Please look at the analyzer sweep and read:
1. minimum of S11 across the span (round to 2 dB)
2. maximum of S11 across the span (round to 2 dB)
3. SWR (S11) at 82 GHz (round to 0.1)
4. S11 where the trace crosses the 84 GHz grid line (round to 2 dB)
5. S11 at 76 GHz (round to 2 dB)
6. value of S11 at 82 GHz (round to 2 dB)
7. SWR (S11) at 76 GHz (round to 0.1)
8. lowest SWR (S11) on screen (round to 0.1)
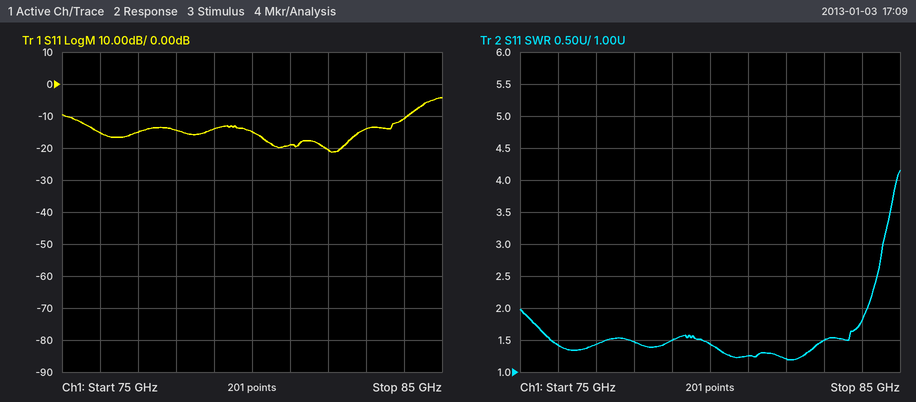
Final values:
-22 dB
-4 dB
1.2
-10 dB
-16 dB
-20 dB
1.4
1.2
